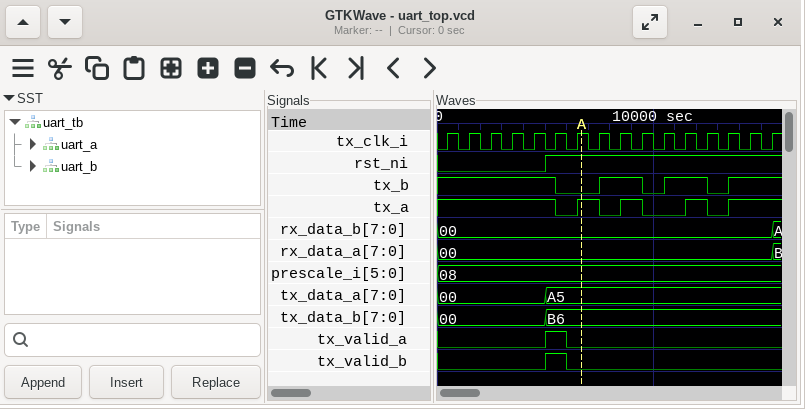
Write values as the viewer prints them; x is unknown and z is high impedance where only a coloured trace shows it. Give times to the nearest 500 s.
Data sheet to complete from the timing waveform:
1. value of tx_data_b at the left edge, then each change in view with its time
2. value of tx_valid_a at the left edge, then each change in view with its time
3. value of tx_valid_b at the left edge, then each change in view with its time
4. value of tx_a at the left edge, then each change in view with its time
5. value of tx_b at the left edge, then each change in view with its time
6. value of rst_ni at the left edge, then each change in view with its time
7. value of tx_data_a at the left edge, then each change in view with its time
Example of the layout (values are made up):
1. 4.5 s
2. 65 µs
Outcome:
1. 00, B6 at 5000 s
2. 0, 1 at 5000 s, 0 at 6000 s
3. 0, 1 at 5000 s, 0 at 6000 s
4. 1, 0 at 5500 s, 1 at 6500 s, 0 at 7500 s, 1 at 8500 s, 0 at 9500 s, 1 at 11500 s, 0 at 12500 s, 1 at 13500 s
5. 1, 0 at 5500 s, 1 at 7500 s, 0 at 9500 s, 1 at 10500 s, 0 at 12500 s, 1 at 13500 s
6. 0, 1 at 5000 s
7. 00, A5 at 5000 s
